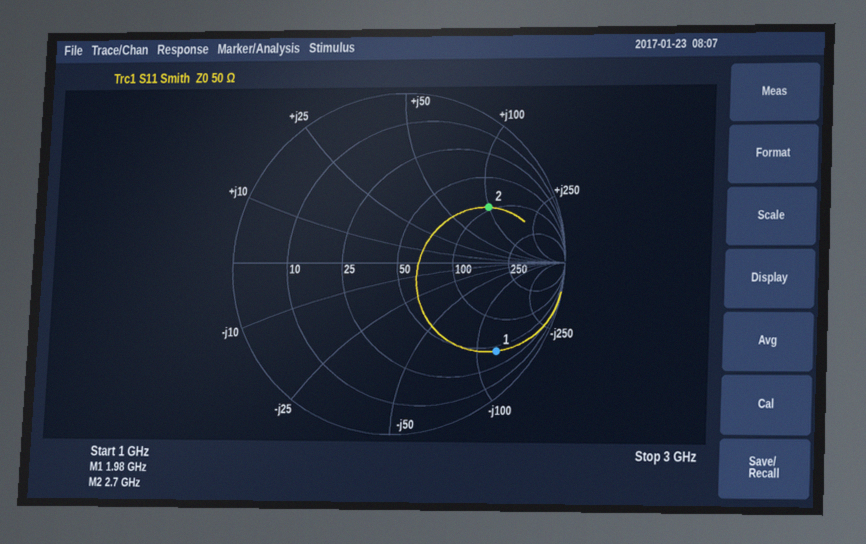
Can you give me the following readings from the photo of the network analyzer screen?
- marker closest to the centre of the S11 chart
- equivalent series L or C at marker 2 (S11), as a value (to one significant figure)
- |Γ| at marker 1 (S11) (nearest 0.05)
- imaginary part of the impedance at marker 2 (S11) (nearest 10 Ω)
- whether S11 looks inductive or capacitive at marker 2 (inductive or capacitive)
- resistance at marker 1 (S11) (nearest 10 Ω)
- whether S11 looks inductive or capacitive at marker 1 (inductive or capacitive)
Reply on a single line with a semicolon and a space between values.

marker 2; 6 nH; 0.80; +100 Ω; inductive; 40 Ω; capacitive
